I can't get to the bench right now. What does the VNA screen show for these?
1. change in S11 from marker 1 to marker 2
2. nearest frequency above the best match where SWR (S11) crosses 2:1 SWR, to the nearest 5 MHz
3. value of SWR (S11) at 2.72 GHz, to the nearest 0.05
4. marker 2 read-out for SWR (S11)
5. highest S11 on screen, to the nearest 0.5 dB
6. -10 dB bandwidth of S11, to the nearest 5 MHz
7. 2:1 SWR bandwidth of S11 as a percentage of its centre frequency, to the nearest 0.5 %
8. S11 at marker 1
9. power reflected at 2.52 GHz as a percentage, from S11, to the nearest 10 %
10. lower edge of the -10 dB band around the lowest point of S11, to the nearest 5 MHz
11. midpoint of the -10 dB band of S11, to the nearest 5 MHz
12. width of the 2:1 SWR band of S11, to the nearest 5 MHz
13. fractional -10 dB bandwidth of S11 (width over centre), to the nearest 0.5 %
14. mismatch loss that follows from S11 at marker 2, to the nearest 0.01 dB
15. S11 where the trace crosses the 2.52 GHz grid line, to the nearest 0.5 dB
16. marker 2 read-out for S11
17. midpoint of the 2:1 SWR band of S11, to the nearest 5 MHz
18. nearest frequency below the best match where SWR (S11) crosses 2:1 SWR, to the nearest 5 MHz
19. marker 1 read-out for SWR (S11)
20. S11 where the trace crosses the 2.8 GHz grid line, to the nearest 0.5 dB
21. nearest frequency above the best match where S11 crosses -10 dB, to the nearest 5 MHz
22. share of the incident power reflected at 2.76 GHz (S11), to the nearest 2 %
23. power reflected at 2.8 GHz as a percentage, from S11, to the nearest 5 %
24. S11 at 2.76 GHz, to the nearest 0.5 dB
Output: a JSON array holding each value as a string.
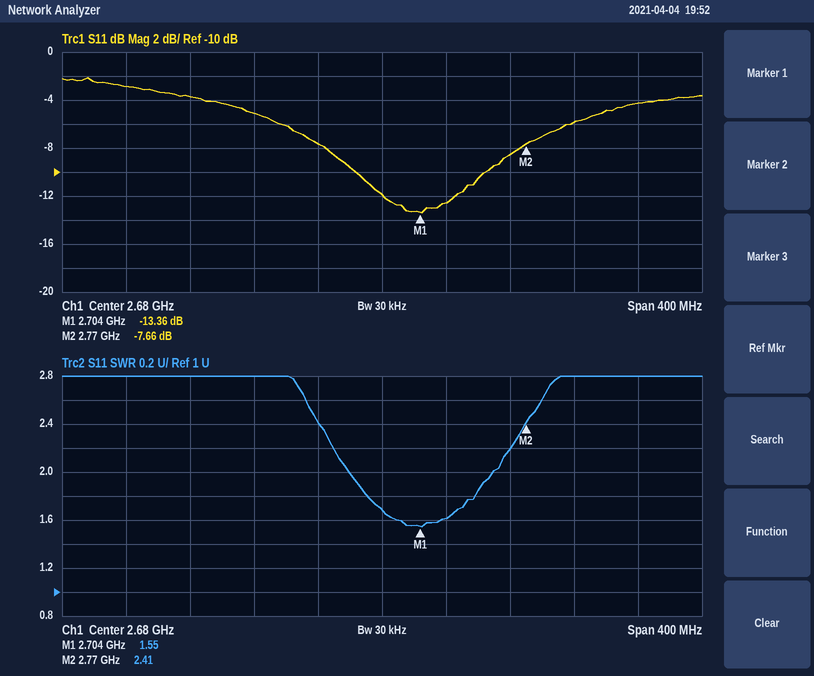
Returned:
["5.70 dB", "2.750 GHz", "1.60", "2.41", "-2.0 dB", "80 MHz", "3.5 %", "-13.36 dB", "50 %", "2.665 GHz", "2.705 GHz", "90 MHz", "3.0 %", "0.82 dB", "-3.0 dB", "-7.66 dB", "2.705 GHz", "2.660 GHz", "1.55", "-6.0 dB", "2.745 GHz", "14 %", "25 %", "-8.5 dB"]
